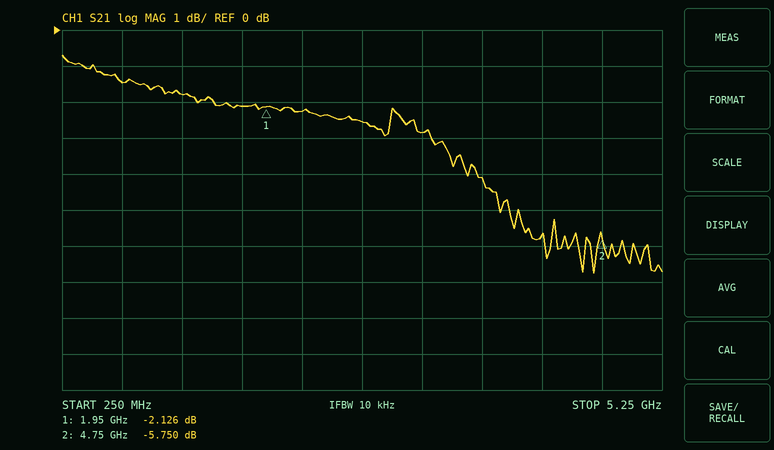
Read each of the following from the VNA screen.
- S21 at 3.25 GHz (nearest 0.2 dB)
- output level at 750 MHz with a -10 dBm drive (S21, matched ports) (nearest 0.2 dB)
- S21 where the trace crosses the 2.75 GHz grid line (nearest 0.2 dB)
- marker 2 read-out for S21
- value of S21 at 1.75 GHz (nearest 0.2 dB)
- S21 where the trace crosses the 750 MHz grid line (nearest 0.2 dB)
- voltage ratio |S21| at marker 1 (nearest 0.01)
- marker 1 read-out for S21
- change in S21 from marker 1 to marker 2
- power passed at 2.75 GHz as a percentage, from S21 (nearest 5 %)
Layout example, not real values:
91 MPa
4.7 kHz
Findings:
-2.8 dB
-11.4 dBm
-2.6 dB
-5.750 dB
-2.2 dB
-1.4 dB
0.78
-2.126 dB
-3.624 dB
55 %
